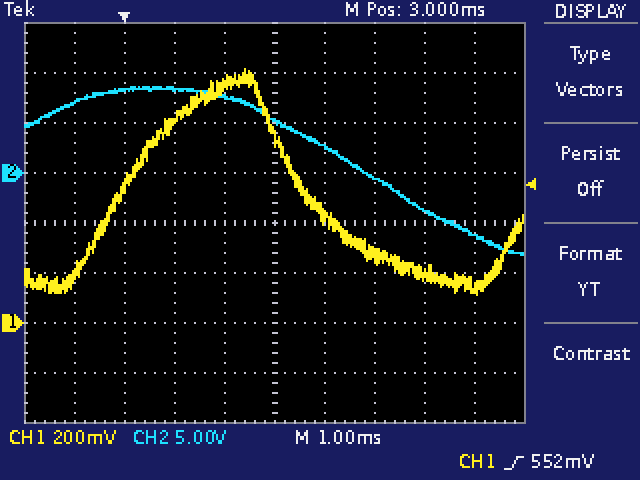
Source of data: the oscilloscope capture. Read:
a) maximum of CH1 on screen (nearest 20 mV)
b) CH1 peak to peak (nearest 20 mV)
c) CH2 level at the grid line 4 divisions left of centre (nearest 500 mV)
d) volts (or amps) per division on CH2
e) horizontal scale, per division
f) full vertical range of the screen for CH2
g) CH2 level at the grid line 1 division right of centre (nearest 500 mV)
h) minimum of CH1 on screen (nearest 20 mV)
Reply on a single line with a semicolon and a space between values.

1.02 V; 900 mV; 7.0 V; 5 V; 1 ms; 40 V; 2.5 V; 120 mV
